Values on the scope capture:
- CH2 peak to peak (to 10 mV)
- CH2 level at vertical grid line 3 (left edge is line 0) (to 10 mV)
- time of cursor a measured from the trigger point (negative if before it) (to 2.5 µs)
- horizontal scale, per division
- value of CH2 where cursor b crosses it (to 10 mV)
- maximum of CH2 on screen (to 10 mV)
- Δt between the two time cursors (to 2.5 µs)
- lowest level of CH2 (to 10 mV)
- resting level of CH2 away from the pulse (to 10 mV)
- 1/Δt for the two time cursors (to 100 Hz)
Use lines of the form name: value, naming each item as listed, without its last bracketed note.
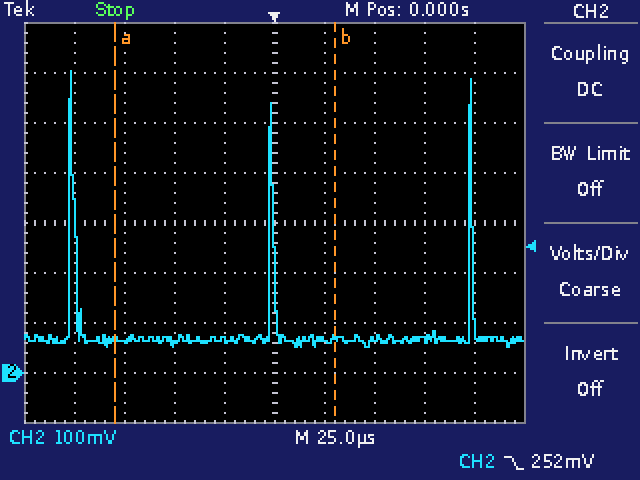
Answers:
CH2 peak to peak: 550 mV
CH2 level at vertical grid line 3 (left edge is line 0): 60 mV
time of cursor a measured from the trigger point (negative if before it): -80.0 µs
horizontal scale, per division: 25 µs
value of CH2 where cursor b crosses it: 70 mV
maximum of CH2 on screen: 600 mV
Δt between the two time cursors: 110.0 µs
lowest level of CH2: 50 mV
resting level of CH2 away from the pulse: 70 mV
1/Δt for the two time cursors: 9.1 kHz
